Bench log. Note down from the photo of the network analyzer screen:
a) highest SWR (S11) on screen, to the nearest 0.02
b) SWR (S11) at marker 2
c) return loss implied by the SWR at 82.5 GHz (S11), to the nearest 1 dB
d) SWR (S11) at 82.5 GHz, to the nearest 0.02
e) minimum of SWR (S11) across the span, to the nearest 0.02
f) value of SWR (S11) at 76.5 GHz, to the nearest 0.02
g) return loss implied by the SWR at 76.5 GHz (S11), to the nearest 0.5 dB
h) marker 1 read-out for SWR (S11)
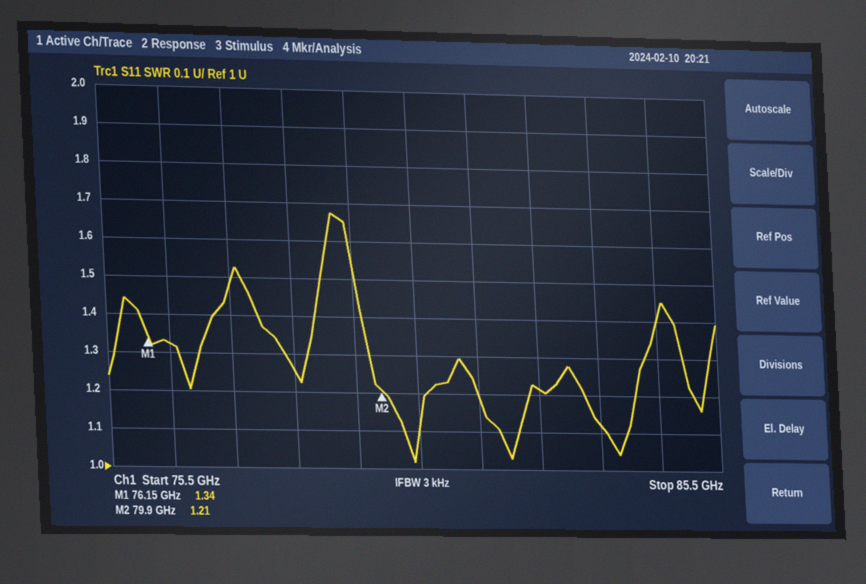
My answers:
1.68
1.21
20 dB
1.22
1.02
1.32
17.0 dB
1.34
